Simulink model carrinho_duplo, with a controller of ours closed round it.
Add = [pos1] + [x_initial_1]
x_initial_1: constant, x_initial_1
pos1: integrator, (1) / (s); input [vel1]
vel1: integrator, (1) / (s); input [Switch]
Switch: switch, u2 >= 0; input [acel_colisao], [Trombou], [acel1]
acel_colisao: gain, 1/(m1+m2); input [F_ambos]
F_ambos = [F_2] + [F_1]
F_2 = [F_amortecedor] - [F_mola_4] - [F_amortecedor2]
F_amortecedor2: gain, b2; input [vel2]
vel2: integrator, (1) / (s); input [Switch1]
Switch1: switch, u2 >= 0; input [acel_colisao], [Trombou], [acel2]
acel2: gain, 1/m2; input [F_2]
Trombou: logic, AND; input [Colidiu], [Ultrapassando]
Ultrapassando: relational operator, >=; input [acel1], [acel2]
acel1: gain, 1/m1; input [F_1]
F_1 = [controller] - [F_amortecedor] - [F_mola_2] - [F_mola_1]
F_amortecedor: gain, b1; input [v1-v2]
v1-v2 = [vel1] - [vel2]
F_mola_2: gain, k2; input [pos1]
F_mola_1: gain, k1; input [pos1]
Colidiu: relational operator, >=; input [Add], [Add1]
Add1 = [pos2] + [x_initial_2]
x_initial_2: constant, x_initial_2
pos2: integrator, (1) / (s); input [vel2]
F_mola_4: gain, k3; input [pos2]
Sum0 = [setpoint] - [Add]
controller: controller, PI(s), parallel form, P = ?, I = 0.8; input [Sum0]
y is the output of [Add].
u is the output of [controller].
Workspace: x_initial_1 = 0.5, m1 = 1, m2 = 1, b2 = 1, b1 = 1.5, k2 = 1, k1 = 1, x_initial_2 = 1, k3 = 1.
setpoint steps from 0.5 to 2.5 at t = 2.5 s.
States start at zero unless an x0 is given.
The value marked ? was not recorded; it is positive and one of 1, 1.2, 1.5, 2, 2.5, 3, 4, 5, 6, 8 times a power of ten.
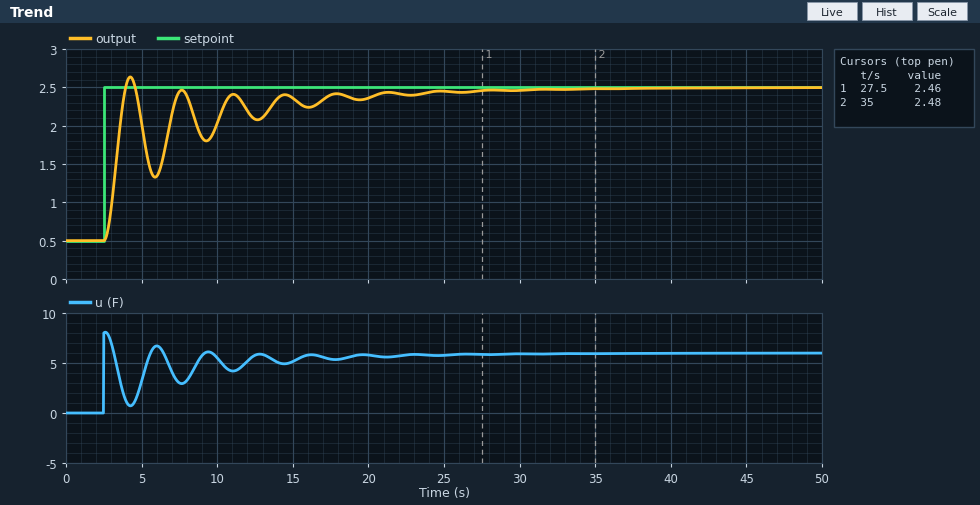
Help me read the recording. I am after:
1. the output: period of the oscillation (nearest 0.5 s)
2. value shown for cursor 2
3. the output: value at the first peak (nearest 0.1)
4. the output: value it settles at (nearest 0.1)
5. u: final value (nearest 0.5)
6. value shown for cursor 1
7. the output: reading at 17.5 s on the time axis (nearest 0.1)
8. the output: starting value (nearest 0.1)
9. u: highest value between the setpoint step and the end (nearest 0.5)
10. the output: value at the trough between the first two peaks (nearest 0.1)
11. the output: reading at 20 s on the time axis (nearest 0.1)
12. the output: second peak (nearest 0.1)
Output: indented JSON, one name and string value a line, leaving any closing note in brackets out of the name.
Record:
{
  "the output: period of the oscillation": "3.5 s",
  "value shown for cursor 2": "2.48",
  "the output: value at the first peak": "2.6",
  "the output: value it settles at": "2.5",
  "u: final value": "6.0",
  "value shown for cursor 1": "2.46",
  "the output: reading at 17.5 s on the time axis": "2.4",
  "the output: starting value": "0.5",
  "u: highest value between the setpoint step and the end": "8.0",
  "the output: value at the trough between the first two peaks": "1.3",
  "the output: reading at 20 s on the time axis": "2.4",
  "the output: second peak": "2.5"
}
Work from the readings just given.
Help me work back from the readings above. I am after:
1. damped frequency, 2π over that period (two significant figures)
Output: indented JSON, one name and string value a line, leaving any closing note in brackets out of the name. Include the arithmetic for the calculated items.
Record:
{
  "damped frequency, 2π over that period": "2π / 3.5 = 1.8 rad/s"
}
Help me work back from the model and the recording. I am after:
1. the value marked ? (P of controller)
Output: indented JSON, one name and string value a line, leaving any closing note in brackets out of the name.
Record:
{
  "the value marked ?": "4"
}
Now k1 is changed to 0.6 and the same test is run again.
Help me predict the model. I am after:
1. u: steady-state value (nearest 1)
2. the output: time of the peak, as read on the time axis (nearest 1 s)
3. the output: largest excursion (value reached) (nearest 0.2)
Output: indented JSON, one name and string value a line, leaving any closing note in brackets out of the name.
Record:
{
  "u: steady-state value": "5",
  "the output: time of the peak, as read on the time axis": "4 s",
  "the output: largest excursion (value reached)": "2.8"
}
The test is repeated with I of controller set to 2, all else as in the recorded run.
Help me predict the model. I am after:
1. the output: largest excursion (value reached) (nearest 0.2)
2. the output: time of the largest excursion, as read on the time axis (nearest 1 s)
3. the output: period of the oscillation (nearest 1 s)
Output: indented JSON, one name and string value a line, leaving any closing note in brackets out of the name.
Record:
{
  "the output: largest excursion (value reached)": "3.0",
  "the output: time of the largest excursion, as read on the time axis": "8 s",
  "the output: period of the oscillation": "3 s"
}
